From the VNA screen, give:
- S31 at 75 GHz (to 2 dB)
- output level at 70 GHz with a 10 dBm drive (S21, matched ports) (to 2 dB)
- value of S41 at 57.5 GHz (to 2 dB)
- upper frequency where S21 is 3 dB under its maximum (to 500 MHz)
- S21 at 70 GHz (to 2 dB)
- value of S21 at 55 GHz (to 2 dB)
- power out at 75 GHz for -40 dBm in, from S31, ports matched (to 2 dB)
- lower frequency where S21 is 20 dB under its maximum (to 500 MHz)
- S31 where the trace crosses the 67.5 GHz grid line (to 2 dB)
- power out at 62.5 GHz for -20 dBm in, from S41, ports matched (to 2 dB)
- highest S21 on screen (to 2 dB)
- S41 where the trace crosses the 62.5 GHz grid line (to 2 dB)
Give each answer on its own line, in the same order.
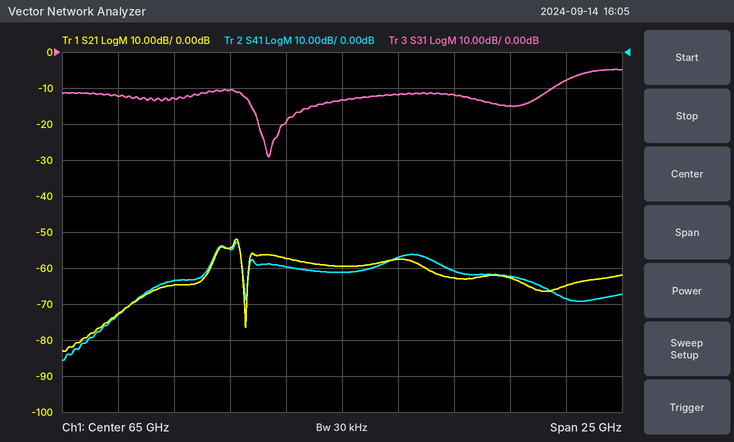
-8 dB
-52 dBm
-64 dB
60.5 GHz
-62 dB
-72 dB
-48 dBm
55.0 GHz
-12 dB
-80 dBm
-52 dB
-60 dB
